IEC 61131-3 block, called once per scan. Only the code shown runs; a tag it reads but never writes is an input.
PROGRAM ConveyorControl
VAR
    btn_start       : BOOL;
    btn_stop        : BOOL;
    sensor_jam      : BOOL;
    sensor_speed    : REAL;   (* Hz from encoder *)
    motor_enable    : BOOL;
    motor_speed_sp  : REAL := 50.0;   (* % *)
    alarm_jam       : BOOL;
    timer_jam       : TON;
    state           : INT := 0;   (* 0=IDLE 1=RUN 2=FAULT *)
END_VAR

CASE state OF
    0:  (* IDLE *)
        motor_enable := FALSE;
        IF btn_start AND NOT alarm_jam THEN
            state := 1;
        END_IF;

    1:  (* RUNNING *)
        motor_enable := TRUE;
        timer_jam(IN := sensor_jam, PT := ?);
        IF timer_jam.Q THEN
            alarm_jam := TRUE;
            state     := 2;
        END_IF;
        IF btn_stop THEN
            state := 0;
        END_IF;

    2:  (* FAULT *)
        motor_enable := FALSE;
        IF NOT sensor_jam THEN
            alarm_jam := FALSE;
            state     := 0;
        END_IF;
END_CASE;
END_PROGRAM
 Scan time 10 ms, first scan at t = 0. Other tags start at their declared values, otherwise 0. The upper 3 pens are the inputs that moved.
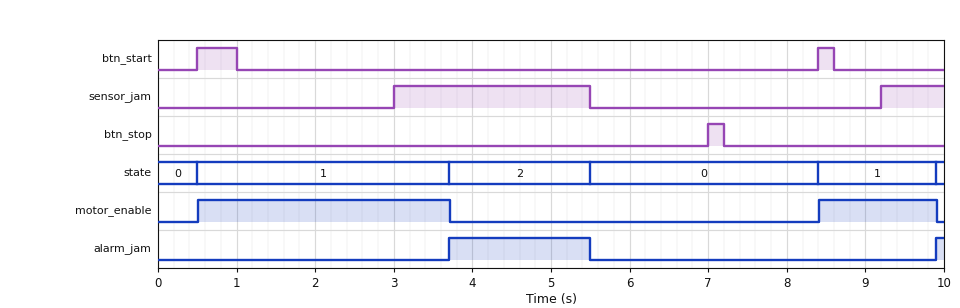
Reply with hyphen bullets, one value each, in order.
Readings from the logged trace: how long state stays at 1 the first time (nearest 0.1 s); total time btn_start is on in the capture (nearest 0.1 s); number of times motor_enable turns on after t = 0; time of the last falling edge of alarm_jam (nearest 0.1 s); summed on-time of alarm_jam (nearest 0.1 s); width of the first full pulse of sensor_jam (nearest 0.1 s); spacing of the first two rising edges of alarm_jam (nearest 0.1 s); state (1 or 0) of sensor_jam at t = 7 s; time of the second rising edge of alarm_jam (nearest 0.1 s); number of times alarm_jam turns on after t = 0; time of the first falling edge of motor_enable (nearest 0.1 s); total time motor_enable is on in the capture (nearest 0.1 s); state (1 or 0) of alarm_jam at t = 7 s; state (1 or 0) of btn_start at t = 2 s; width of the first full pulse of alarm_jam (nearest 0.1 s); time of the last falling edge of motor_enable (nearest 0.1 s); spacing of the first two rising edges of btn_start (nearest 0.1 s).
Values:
- 3.2 s
- 0.7 s
- 2
- 5.5 s
- 1.9 s
- 2.5 s
- 6.2 s
- 0
- 9.9 s
- 2
- 3.7 s
- 4.7 s
- 0
- 0
- 1.8 s
- 9.9 s
- 7.9 s
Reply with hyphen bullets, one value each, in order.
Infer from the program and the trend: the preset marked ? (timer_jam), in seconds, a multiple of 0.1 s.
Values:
- 0.7 s
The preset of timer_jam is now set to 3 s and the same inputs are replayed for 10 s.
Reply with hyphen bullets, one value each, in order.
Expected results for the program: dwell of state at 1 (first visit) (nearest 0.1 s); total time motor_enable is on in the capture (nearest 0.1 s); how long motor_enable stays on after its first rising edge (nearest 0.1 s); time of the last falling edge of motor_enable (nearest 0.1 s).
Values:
- 6.5 s
- 8.1 s
- 6.5 s
- 7.0 s
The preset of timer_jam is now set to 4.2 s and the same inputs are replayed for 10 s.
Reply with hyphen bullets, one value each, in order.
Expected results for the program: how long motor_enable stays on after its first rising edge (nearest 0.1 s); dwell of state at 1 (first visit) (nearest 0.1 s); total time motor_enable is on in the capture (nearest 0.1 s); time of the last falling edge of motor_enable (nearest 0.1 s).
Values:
- 6.5 s
- 6.5 s
- 8.1 s
- 7.0 s
